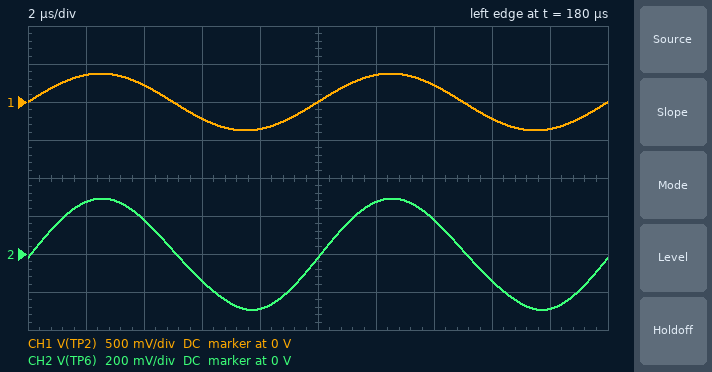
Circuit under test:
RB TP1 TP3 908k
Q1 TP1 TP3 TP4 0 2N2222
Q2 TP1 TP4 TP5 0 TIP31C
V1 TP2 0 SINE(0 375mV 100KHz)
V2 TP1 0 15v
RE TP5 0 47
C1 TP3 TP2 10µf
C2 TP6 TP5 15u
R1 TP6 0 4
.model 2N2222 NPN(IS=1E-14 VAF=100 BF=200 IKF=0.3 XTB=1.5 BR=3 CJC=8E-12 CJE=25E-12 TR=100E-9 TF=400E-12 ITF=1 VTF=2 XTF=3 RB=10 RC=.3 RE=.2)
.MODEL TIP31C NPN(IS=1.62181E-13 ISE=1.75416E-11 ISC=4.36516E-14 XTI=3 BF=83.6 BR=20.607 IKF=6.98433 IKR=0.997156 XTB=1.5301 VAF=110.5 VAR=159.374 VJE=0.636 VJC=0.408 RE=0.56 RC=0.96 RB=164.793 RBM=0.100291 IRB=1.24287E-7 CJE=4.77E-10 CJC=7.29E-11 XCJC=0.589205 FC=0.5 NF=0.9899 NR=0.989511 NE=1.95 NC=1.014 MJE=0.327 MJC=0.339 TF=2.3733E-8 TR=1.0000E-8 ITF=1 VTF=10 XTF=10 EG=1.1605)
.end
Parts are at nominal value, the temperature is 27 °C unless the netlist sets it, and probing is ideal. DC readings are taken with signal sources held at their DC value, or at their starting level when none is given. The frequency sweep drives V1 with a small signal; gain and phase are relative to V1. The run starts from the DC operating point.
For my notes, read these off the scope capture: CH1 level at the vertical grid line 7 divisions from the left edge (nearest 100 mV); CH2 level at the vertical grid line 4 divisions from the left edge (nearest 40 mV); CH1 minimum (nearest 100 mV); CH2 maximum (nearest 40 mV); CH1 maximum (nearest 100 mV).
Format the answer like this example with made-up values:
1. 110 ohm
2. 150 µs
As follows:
1. 200 mV
2. -280 mV
3. -400 mV
4. 280 mV
5. 400 mV
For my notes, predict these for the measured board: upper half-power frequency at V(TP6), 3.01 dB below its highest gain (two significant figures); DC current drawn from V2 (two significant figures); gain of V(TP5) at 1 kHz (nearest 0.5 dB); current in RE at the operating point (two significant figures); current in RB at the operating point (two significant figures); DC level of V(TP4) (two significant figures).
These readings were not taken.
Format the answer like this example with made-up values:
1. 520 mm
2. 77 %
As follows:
1. 1.2 MHz
2. 140 mA
3. -0.5 dB
4. 140 mA
5. 7.6 µA
6. 7.4 V
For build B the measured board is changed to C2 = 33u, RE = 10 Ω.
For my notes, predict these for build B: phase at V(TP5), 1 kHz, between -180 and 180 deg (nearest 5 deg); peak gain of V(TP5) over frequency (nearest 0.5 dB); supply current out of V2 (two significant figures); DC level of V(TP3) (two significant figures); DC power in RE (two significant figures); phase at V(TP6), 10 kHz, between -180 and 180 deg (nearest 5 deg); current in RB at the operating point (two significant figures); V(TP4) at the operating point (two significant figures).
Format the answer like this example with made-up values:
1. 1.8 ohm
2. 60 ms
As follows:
1. -5 deg
2. -0.5 dB
3. 240 mA
4. 3.9 V
5. 580 mW
6. 5 deg
7. 12 µA
8. 3.3 V
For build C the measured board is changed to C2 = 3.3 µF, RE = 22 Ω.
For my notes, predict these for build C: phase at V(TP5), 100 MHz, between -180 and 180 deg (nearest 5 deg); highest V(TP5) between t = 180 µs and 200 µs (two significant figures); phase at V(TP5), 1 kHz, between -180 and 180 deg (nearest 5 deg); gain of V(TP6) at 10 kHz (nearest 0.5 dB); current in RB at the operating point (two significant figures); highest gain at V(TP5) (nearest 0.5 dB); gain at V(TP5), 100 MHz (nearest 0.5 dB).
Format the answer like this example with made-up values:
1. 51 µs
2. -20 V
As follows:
1. -5 deg
2. 4.6 V
3. 0 deg
4. -5.0 dB
5. 10 µA
6. -0.5 dB
7. -14.0 dB
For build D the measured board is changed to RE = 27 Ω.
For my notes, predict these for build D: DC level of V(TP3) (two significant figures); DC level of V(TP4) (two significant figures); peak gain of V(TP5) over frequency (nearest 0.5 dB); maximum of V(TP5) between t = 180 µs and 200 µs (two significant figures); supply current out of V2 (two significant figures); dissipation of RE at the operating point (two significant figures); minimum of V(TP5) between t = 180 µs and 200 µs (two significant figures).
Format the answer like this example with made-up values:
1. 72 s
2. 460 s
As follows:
1. 6.4 V
2. 5.7 V
3. -0.5 dB
4. 5.2 V
5. 180 mA
6. 890 mW
7. 4.6 V
